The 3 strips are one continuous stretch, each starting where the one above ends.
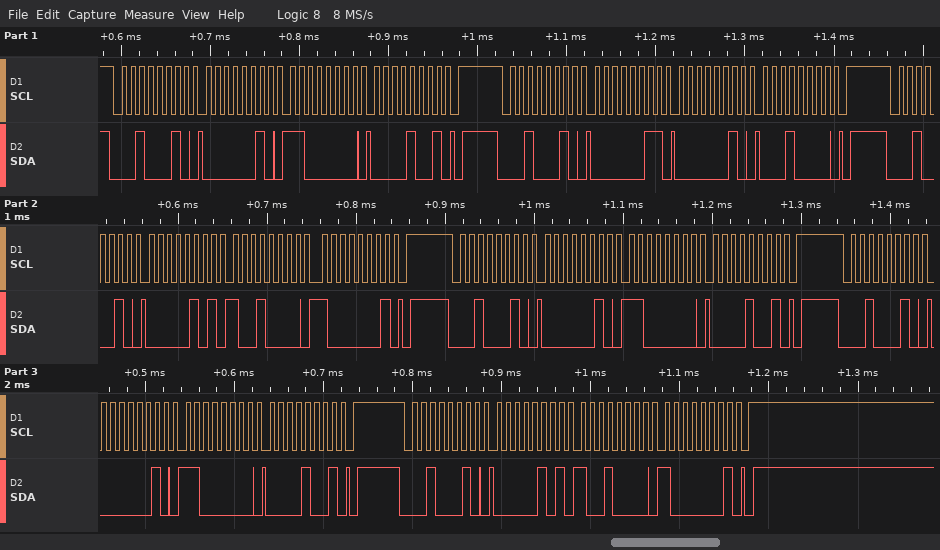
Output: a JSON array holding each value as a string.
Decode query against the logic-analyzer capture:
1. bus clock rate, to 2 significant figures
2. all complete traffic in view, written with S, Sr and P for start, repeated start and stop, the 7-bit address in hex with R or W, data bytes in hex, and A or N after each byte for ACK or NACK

["100 kHz", "S 11W A 02 A C0 A 09 A P S 11W A 03 A 02 A 10 A P S 11W A 05 A 90 A 81 A P S 11W A 02 A C0 A 09 A P S 11W A 02 A C0 A 09 A P S 11W A 05 A 90 A 81 A P"]
